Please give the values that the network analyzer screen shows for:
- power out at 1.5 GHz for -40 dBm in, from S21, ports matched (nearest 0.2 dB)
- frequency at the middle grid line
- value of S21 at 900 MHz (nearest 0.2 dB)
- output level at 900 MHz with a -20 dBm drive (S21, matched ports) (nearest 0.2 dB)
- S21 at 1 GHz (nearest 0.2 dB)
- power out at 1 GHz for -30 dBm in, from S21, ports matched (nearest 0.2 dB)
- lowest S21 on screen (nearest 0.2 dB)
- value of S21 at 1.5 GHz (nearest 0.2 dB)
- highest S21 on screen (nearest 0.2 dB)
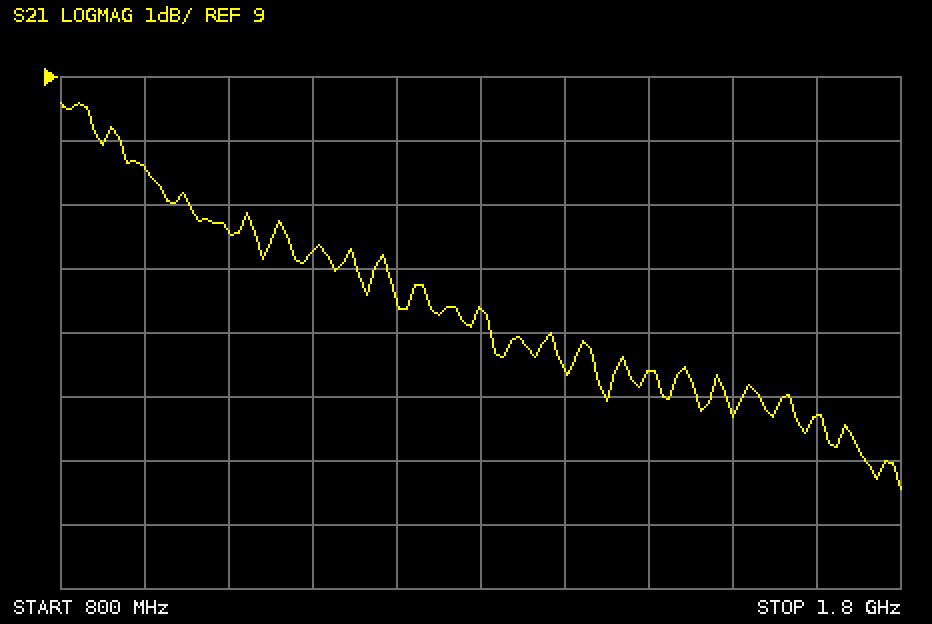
-35.6 dBm
1.3 GHz
7.6 dB
-12.4 dBm
6.6 dB
-23.4 dBm
2.6 dB
4.4 dB
8.6 dB
